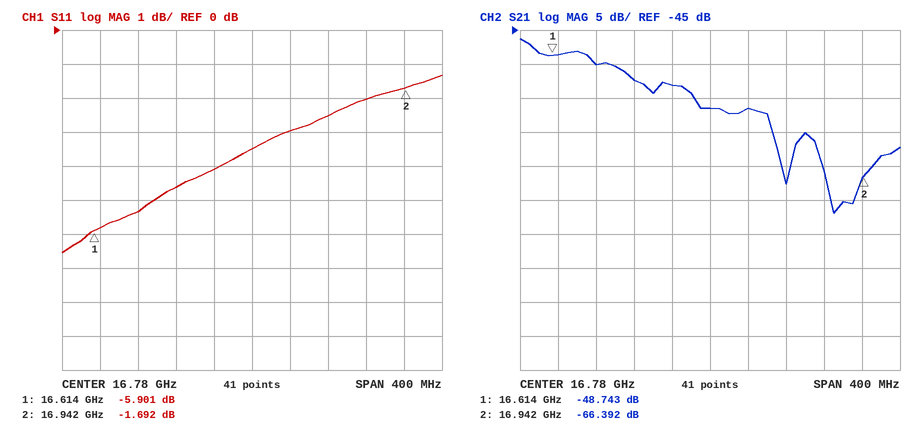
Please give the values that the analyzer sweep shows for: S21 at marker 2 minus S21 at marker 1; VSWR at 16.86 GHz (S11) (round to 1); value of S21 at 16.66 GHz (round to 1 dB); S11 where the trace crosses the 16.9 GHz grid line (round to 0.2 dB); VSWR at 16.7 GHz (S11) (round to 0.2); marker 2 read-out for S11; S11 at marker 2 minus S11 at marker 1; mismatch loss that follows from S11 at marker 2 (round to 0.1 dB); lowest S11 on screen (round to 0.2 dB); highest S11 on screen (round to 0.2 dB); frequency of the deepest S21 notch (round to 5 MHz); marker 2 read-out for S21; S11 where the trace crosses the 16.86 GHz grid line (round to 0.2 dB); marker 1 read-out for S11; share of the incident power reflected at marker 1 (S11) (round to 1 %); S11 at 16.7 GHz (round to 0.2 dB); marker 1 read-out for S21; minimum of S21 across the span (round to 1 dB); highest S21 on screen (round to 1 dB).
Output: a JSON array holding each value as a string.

["-17.649 dB", "7", "-50 dB", "-2.0 dB", "3.8", "-1.692 dB", "4.209 dB", "4.9 dB", "-6.6 dB", "-1.4 dB", "16.910 GHz", "-66.392 dB", "-2.6 dB", "-5.901 dB", "26 %", "-4.6 dB", "-48.743 dB", "-72 dB", "-46 dB"]
